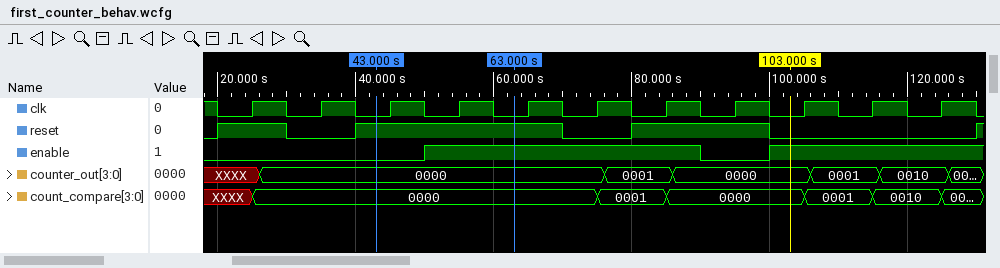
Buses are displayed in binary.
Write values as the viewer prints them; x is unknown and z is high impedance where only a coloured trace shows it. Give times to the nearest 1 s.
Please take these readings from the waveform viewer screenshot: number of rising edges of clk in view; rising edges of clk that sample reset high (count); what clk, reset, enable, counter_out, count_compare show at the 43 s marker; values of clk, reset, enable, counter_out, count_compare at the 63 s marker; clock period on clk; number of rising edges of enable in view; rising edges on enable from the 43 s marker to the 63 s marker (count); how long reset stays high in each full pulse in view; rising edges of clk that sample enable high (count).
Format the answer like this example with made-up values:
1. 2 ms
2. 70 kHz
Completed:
1. 11
2. 6
3. clk=0, reset=1, enable=0, counter_out=0000, count_compare=0000
4. clk=0, reset=1, enable=1, counter_out=0000, count_compare=0000
5. 10 s
6. 2
7. 1
8. 10 s, 30 s, 20 s
9. 7
